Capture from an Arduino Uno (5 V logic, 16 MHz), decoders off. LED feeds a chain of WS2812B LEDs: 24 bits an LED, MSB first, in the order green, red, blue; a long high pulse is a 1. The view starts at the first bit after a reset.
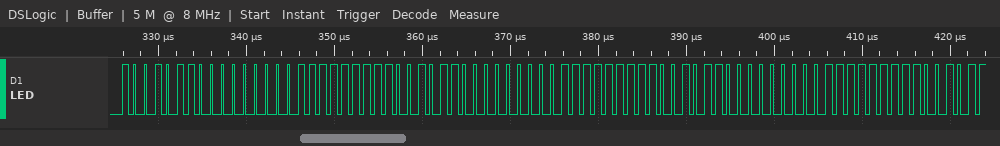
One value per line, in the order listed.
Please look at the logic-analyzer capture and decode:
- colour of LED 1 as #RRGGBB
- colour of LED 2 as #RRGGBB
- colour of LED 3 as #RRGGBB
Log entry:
#0096FF
#0096FF
#0096FF
